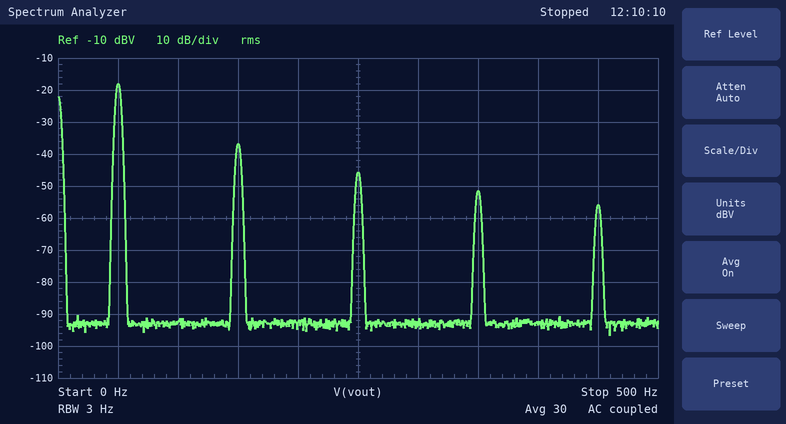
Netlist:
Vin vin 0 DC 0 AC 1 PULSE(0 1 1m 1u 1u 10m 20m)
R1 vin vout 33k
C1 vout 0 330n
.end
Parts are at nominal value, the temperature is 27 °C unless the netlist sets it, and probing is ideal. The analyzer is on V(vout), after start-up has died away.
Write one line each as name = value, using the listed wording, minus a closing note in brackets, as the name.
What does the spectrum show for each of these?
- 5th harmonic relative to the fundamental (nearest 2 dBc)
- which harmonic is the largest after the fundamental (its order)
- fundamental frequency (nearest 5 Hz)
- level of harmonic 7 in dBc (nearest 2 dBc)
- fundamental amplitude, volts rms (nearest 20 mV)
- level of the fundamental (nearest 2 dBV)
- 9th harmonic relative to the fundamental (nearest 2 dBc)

5th harmonic relative to the fundamental = -28 dBc
which harmonic is the largest after the fundamental = 3
fundamental frequency = 50 Hz
level of harmonic 7 in dBc = -34 dBc
fundamental amplitude, volts rms = 120 mV
level of the fundamental = -18 dBV
9th harmonic relative to the fundamental = -38 dBc
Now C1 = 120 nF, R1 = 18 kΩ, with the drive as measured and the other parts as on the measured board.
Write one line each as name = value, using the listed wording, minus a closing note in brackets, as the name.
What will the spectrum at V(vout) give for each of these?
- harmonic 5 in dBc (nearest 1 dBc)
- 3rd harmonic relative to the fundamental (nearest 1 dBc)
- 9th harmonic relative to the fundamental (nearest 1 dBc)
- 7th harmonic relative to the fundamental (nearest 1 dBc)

harmonic 5 in dBc = -23 dBc
3rd harmonic relative to the fundamental = -15 dBc
9th harmonic relative to the fundamental = -33 dBc
7th harmonic relative to the fundamental = -29 dBc
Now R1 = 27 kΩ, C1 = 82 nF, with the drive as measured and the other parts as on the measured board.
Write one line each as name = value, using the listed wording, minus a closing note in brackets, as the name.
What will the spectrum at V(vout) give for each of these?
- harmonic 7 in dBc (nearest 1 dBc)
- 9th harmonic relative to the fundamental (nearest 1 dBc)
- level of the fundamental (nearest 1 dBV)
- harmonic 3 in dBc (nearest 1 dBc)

harmonic 7 in dBc = -29 dBc
9th harmonic relative to the fundamental = -33 dBc
level of the fundamental = -9 dBV
harmonic 3 in dBc = -15 dBc
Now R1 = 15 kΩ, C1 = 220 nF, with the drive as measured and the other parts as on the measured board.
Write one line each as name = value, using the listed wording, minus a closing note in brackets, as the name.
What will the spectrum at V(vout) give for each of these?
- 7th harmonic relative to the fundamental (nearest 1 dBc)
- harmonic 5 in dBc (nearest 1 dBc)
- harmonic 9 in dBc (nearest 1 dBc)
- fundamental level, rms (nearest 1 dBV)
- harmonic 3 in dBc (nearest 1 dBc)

7th harmonic relative to the fundamental = -31 dBc
harmonic 5 in dBc = -25 dBc
harmonic 9 in dBc = -35 dBc
fundamental level, rms = -10 dBV
harmonic 3 in dBc = -17 dBc
